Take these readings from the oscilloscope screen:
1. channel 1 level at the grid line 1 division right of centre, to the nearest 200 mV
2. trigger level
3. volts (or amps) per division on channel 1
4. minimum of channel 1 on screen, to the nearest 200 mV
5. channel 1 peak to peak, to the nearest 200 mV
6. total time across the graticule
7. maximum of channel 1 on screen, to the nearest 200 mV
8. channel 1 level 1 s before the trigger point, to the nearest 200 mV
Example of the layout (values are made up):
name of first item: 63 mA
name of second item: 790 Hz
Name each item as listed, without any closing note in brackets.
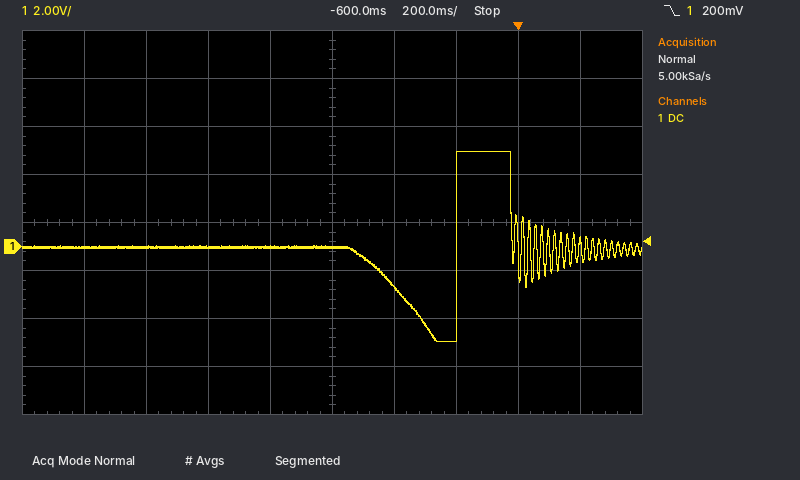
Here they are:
channel 1 level at the grid line 1 division right of centre, to the nearest 200 mV: -1.6 V
trigger level: 200 mV
volts (or amps) per division on channel 1: 2 V
minimum of channel 1 on screen, to the nearest 200 mV: -4.0 V
channel 1 peak to peak, to the nearest 200 mV: 8.0 V
total time across the graticule: 2 s
maximum of channel 1 on screen, to the nearest 200 mV: 4.0 V
channel 1 level 1 s before the trigger point, to the nearest 200 mV: 0.0 V
